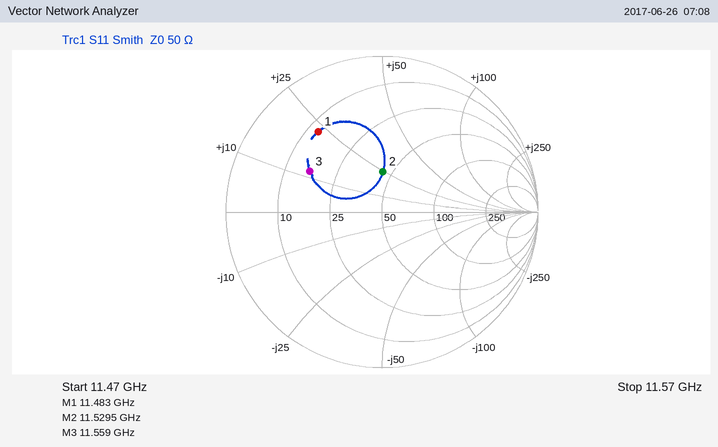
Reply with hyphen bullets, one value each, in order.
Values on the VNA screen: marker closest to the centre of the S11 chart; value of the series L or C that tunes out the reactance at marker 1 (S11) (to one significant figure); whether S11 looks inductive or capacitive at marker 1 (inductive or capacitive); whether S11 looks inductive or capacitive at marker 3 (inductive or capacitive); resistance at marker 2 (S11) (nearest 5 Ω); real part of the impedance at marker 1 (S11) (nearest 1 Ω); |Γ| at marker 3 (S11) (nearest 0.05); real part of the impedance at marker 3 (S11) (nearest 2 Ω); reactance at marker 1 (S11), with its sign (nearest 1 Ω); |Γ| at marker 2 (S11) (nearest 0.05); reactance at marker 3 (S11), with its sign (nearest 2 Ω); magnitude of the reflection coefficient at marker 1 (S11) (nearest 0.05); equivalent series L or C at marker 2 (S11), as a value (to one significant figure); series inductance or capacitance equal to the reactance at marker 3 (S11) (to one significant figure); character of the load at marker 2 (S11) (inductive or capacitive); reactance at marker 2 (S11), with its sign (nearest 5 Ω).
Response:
- marker 2
- 600 fF
- inductive
- inductive
- 45 Ω
- 13 Ω
- 0.55
- 16 Ω
- +23 Ω
- 0.25
- +12 Ω
- 0.65
- 300 pH
- 200 pH
- inductive
- +25 Ω
